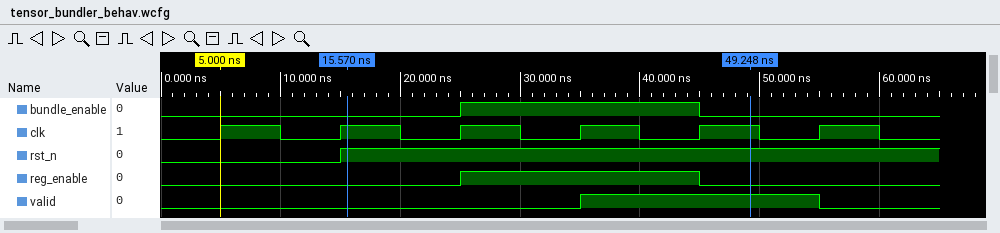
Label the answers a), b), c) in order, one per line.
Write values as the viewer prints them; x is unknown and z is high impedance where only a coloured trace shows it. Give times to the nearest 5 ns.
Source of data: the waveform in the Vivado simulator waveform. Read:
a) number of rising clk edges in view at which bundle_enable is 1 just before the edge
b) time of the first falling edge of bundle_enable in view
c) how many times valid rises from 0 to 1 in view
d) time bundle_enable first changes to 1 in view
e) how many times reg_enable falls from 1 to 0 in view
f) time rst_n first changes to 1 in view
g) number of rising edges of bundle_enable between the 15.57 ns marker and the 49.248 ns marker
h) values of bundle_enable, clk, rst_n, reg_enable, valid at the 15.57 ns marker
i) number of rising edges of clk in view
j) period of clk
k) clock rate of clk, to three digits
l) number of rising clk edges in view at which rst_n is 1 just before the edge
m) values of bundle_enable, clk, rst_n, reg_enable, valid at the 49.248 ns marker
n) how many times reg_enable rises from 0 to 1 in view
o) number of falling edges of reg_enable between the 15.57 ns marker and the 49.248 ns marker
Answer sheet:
a) 2
b) 45 ns
c) 1
d) 25 ns
e) 1
f) 15 ns
g) 1
h) bundle_enable=0, clk=1, rst_n=1, reg_enable=0, valid=0
i) 6
j) 10 ns
k) 100 MHz
l) 4
m) bundle_enable=0, clk=1, rst_n=1, reg_enable=0, valid=1
n) 1
o) 1
